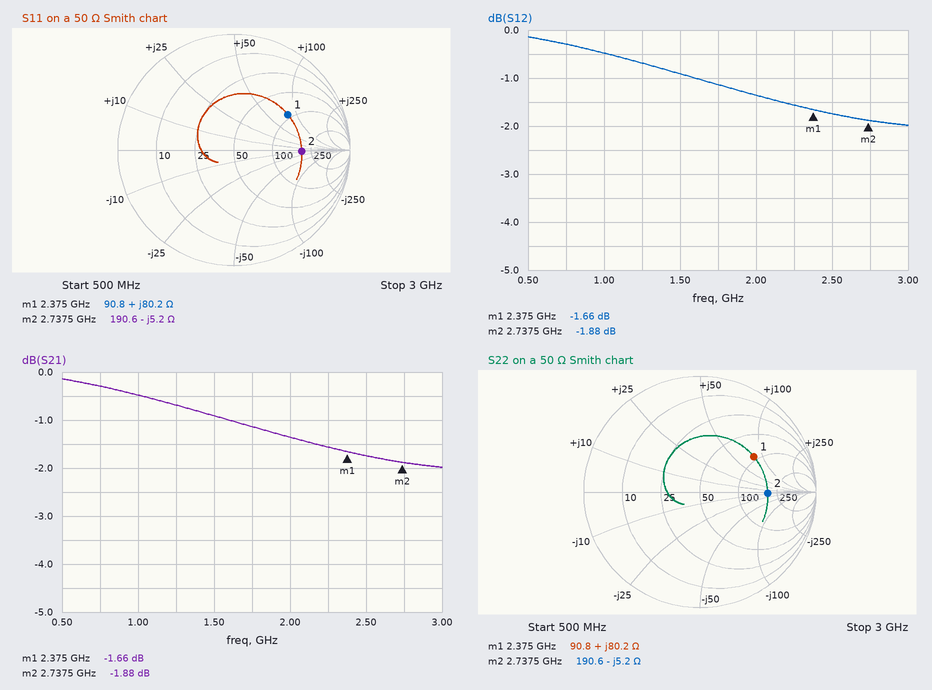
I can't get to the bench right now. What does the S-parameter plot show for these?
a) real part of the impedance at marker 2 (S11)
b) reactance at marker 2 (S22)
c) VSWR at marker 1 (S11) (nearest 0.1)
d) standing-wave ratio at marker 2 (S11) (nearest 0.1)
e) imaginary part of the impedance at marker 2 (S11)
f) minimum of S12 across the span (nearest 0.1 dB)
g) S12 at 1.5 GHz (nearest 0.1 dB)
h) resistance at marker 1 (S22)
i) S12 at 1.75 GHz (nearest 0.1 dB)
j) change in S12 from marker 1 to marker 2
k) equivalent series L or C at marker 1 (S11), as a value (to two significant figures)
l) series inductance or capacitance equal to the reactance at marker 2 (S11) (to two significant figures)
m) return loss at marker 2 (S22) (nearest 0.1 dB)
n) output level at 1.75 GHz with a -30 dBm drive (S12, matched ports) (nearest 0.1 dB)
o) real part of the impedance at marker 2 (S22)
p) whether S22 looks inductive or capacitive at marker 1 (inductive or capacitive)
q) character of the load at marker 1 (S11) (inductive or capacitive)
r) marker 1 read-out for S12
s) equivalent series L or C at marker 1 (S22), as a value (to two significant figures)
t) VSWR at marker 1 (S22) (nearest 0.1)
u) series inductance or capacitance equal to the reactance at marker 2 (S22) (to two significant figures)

190.6 Ω
-5.2 Ω
3.5
3.8
-5.2 Ω
-2.0 dB
-0.9 dB
90.8 Ω
-1.1 dB
-0.22 dB
5.4 nH
11 pF
4.7 dB
-31.1 dBm
190.6 Ω
inductive
inductive
-1.66 dB
5.4 nH
3.5
11 pF
